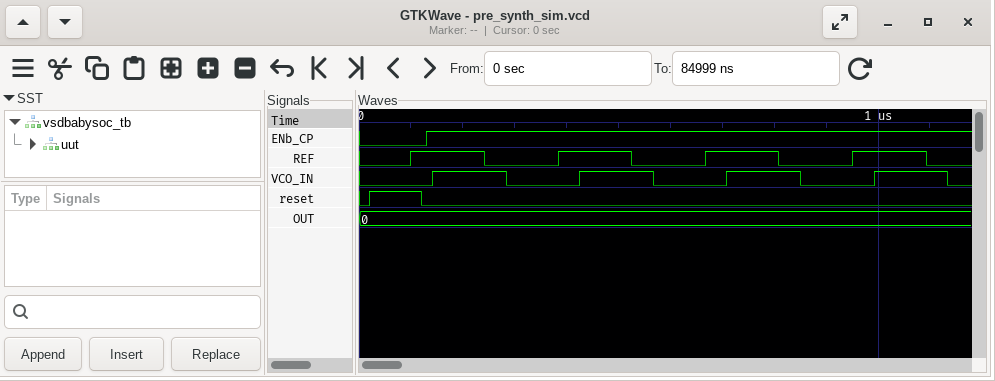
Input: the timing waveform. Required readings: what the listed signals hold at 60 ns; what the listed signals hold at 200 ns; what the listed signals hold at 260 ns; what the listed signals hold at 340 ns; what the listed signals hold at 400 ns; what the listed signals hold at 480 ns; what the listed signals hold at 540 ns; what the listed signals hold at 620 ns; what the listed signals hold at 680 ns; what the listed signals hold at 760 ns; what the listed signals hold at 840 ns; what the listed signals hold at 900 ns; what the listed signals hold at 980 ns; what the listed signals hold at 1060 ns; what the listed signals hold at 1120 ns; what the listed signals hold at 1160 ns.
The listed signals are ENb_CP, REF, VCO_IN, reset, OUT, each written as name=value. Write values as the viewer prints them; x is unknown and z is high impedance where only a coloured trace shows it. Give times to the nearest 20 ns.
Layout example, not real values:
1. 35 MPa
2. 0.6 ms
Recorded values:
1. ENb_CP=0, REF=0, VCO_IN=0, reset=1, OUT=0
2. ENb_CP=1, REF=1, VCO_IN=1, reset=0, OUT=0
3. ENb_CP=1, REF=0, VCO_IN=1, reset=0, OUT=0
4. ENb_CP=1, REF=0, VCO_IN=0, reset=0, OUT=0
5. ENb_CP=1, REF=1, VCO_IN=0, reset=0, OUT=0
6. ENb_CP=1, REF=1, VCO_IN=1, reset=0, OUT=0
7. ENb_CP=1, REF=0, VCO_IN=1, reset=0, OUT=0
8. ENb_CP=1, REF=0, VCO_IN=0, reset=0, OUT=0
9. ENb_CP=1, REF=1, VCO_IN=0, reset=0, OUT=0
10. ENb_CP=1, REF=1, VCO_IN=1, reset=0, OUT=0
11. ENb_CP=1, REF=0, VCO_IN=1, reset=0, OUT=0
12. ENb_CP=1, REF=0, VCO_IN=0, reset=0, OUT=0
13. ENb_CP=1, REF=1, VCO_IN=0, reset=0, OUT=0
14. ENb_CP=1, REF=1, VCO_IN=1, reset=0, OUT=0
15. ENb_CP=1, REF=0, VCO_IN=1, reset=0, OUT=0
16. ENb_CP=1, REF=0, VCO_IN=0, reset=0, OUT=0
